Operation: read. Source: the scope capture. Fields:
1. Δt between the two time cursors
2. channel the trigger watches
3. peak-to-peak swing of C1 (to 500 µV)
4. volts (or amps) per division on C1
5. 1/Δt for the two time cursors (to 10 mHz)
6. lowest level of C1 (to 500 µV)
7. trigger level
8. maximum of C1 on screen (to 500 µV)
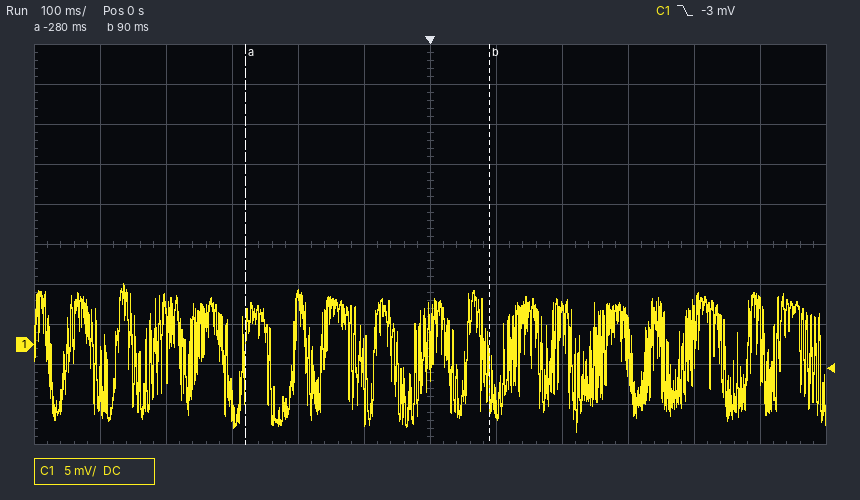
370 ms
C1
18.5 mV
5 mV
2.70 Hz
-11.0 mV
-3 mV
7.5 mV
